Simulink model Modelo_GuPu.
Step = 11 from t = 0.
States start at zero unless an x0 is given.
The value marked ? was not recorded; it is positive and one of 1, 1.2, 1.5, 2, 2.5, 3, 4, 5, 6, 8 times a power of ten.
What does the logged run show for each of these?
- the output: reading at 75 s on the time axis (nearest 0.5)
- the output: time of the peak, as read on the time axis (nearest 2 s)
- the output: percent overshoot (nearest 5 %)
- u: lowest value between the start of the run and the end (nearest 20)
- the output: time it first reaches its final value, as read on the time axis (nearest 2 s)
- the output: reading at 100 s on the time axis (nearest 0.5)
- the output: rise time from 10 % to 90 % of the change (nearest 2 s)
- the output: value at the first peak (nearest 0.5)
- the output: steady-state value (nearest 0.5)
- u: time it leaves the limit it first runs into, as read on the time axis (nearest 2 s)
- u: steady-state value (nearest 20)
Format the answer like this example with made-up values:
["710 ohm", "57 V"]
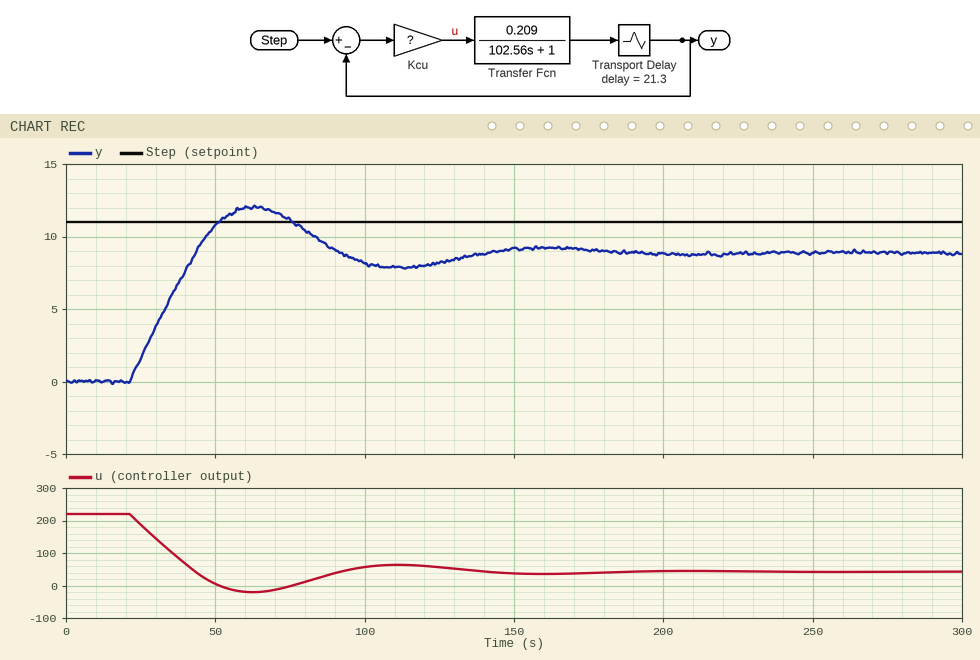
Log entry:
["11.0", "62 s", "35 %", "-20", "44 s", "8.0", "18 s", "12.0", "9.0", "22 s", "40"]
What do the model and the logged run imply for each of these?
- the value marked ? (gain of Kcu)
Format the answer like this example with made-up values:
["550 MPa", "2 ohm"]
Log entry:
["20"]
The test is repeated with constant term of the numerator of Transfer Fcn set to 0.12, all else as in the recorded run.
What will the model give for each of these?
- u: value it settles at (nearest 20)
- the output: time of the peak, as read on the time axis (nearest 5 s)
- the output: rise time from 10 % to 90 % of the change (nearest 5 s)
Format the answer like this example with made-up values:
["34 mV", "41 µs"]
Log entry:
["60", "80 s", "30 s"]
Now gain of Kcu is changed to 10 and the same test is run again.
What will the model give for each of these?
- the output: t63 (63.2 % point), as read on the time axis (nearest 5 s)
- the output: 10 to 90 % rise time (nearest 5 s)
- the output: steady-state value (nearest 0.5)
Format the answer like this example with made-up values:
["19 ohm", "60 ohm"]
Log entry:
["45 s", "35 s", "7.5"]
